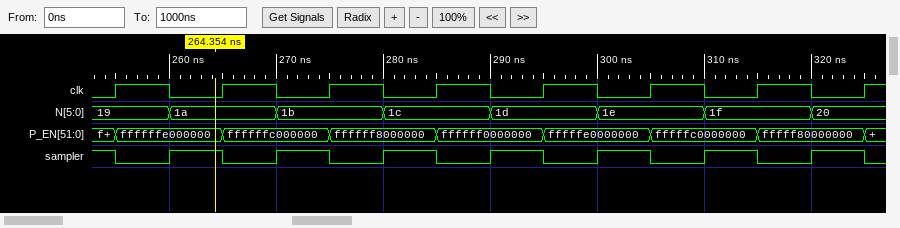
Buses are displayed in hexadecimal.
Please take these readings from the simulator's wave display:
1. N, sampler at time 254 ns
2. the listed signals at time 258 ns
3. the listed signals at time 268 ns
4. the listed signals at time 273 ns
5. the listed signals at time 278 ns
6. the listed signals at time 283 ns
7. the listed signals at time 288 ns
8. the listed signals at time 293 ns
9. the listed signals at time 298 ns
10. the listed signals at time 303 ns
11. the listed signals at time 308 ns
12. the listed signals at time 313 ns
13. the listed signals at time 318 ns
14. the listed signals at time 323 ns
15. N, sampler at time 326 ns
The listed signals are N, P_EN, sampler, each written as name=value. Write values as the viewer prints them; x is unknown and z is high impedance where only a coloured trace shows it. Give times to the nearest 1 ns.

N=19, sampler=1
N=19, P_EN=ffffffe000000, sampler=0
N=1a, P_EN=ffffffc000000, sampler=0
N=1b, P_EN=ffffffc000000, sampler=1
N=1b, P_EN=ffffff8000000, sampler=0
N=1c, P_EN=ffffff8000000, sampler=1
N=1c, P_EN=ffffff0000000, sampler=0
N=1d, P_EN=ffffff0000000, sampler=1
N=1d, P_EN=fffffe0000000, sampler=0
N=1e, P_EN=fffffe0000000, sampler=1
N=1e, P_EN=fffffc0000000, sampler=0
N=1f, P_EN=fffffc0000000, sampler=1
N=1f, P_EN=fffff80000000, sampler=0
N=20, P_EN=fffff80000000, sampler=1
N=20, sampler=0
